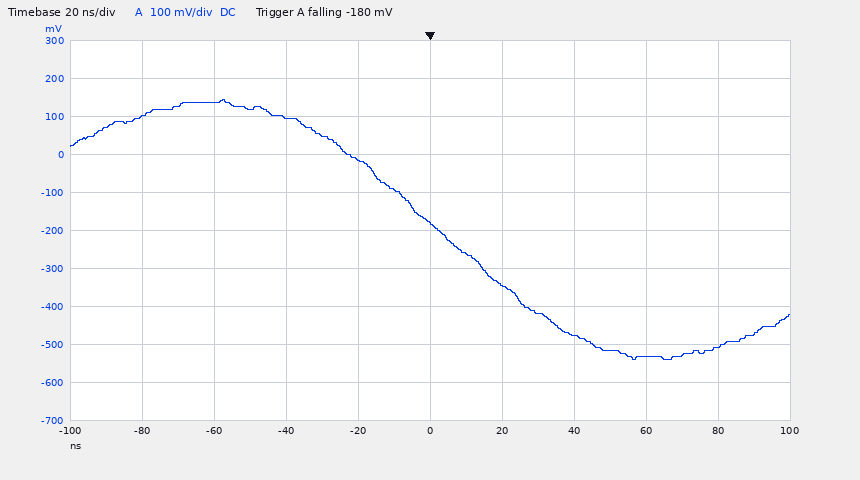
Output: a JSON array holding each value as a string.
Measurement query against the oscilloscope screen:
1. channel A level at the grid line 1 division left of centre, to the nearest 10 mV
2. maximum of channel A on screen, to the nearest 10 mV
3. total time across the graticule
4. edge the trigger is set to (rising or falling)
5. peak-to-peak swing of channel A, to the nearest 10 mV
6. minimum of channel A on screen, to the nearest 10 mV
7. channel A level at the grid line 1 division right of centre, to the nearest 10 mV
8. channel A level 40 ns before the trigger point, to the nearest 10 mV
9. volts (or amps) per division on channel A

["-10 mV", "140 mV", "200 ns", "falling", "680 mV", "-540 mV", "-340 mV", "100 mV", "100 mV"]
